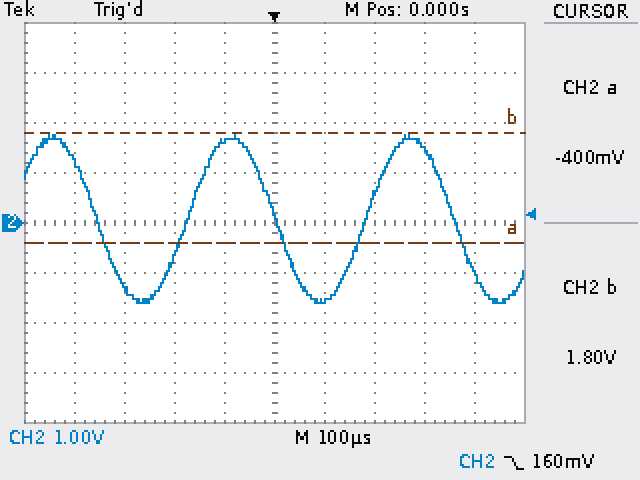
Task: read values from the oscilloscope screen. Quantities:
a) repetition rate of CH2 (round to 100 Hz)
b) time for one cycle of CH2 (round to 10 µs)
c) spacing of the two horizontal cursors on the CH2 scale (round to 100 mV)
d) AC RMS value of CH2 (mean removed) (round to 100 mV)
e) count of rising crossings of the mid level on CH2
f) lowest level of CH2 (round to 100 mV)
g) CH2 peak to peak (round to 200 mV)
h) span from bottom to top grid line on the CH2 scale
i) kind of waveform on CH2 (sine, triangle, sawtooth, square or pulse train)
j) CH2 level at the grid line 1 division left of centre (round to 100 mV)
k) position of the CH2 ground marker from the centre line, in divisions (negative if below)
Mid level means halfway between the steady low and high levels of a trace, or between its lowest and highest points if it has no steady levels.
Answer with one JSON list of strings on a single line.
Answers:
["2.8 kHz", "360 µs", "2.2 V", "1.2 V", "2", "-1.6 V", "3.4 V", "8 V", "sine", "1.6 V", "0.0 div"]
